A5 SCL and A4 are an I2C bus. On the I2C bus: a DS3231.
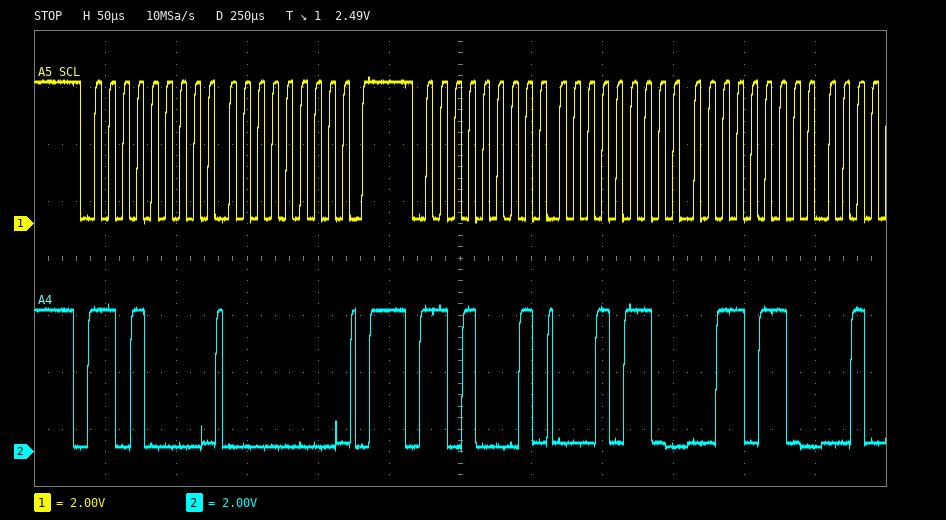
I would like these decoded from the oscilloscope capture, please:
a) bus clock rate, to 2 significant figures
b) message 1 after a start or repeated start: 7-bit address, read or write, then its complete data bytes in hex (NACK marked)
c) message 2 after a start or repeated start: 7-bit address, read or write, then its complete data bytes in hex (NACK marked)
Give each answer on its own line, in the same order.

100 kHz
0x68 write: 00
0x68 read: 16 36
